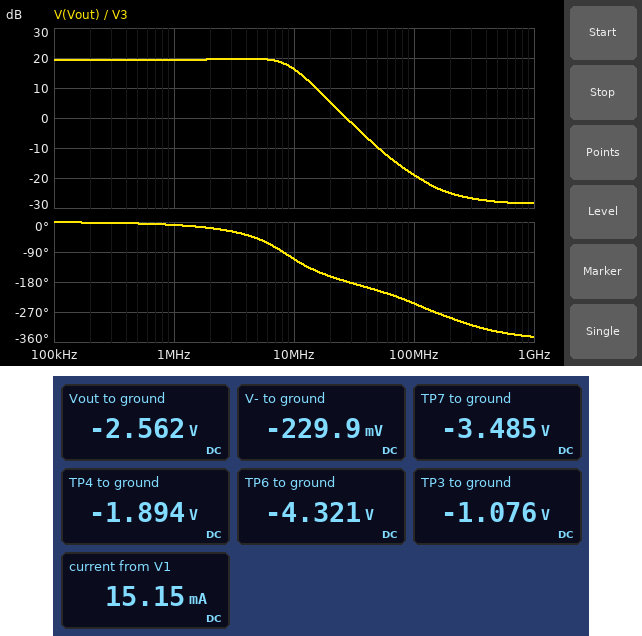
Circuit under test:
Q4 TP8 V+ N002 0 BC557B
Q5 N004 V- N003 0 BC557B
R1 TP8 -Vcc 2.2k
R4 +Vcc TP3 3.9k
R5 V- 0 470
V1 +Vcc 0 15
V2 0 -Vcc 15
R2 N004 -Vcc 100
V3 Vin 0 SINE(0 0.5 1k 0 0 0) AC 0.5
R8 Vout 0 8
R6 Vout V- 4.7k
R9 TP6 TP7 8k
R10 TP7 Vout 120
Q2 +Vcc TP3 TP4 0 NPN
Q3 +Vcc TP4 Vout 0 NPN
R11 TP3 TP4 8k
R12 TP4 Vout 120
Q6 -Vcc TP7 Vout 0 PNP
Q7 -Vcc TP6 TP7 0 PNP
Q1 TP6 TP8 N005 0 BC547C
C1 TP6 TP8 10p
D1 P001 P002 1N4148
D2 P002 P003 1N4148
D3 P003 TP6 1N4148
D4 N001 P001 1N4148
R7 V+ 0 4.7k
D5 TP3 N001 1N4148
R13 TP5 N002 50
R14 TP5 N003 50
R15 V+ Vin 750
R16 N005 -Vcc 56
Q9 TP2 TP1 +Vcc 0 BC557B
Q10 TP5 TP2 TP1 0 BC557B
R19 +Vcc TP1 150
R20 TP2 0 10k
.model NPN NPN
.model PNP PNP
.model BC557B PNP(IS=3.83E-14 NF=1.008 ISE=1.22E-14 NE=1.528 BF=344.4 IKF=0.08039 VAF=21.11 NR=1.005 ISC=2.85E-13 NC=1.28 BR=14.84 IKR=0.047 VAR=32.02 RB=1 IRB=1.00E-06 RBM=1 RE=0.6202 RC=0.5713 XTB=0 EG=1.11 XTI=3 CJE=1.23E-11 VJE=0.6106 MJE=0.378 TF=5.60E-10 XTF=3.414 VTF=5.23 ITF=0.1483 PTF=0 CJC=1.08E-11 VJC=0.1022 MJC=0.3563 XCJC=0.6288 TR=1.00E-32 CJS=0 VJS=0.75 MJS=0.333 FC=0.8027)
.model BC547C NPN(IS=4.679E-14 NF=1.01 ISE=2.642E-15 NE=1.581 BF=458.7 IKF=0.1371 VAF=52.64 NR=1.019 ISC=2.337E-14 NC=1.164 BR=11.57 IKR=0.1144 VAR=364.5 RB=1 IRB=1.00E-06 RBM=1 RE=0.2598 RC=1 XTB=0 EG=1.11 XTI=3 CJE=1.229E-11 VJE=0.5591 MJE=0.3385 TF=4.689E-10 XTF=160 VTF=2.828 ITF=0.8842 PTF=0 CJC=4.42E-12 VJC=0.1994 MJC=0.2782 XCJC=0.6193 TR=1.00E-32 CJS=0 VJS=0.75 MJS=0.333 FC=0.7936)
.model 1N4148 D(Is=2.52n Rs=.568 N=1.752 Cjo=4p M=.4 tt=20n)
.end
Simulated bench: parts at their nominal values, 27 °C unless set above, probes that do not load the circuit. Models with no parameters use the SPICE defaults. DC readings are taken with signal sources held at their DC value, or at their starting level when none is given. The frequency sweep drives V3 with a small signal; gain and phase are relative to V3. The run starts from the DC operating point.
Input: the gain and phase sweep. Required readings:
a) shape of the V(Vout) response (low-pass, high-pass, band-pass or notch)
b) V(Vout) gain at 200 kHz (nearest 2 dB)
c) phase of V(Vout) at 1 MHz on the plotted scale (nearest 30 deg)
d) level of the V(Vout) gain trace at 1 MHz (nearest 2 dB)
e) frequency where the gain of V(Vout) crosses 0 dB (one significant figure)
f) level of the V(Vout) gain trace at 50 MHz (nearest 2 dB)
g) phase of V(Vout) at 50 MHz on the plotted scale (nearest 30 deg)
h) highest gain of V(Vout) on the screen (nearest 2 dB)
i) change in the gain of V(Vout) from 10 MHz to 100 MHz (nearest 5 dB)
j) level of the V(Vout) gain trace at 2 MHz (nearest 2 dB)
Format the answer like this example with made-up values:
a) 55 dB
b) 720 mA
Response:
a) low-pass
b) 20 dB
c) 0 deg
d) 20 dB
e) 30 MHz
f) -10 dB
g) -210 deg
h) 20 dB
i) -35 dB
j) 20 dB
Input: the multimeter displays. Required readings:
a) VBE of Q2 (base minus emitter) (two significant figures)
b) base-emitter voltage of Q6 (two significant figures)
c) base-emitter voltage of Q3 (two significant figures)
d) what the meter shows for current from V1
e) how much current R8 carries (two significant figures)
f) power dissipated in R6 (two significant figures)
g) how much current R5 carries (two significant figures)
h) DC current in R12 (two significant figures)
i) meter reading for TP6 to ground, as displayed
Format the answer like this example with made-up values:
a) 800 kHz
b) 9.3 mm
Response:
a) 820 mV
b) -920 mV
c) 670 mV
d) 15.15 mA
e) 320 mA
f) 1.2 mW
g) 490 µA
h) 5.6 mA
i) -4.321 V
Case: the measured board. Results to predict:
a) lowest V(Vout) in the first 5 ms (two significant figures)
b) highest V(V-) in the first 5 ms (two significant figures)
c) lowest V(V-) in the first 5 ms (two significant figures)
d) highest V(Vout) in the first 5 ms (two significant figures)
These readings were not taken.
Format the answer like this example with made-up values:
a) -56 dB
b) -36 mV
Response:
a) -7.2 V
b) 190 mV
c) -650 mV
d) 2.1 V
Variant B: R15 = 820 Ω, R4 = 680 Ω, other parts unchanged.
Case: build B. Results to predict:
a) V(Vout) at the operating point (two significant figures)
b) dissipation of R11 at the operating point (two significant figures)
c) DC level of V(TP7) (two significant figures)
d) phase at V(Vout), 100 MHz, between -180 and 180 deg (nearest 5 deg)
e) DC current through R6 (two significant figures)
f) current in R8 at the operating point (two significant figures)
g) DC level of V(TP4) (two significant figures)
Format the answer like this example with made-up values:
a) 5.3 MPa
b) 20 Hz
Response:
a) -1.7 V
b) 93 µW
c) -2.7 V
d) 125 deg
e) 330 µA
f) 210 mA
g) -720 mV
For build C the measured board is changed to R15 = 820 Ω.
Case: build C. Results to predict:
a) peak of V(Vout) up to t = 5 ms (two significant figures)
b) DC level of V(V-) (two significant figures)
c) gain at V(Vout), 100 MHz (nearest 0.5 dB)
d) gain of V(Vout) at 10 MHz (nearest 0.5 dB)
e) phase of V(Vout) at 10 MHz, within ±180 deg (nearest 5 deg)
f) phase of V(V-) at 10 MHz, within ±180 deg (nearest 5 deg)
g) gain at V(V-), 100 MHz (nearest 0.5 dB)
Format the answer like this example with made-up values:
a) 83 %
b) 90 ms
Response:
a) 2.0 V
b) -230 mV
c) -19.5 dB
d) 16.0 dB
e) -115 deg
f) -120 deg
g) -14.0 dB
